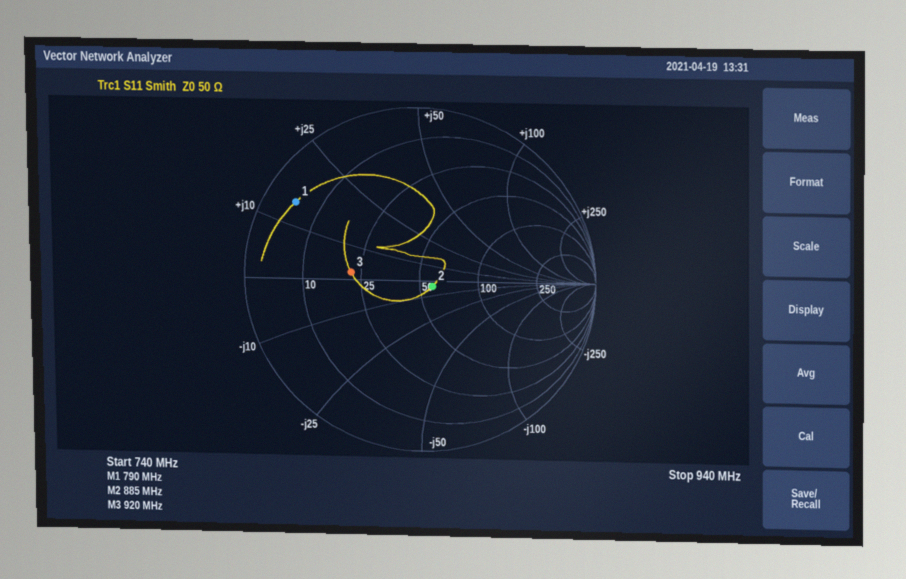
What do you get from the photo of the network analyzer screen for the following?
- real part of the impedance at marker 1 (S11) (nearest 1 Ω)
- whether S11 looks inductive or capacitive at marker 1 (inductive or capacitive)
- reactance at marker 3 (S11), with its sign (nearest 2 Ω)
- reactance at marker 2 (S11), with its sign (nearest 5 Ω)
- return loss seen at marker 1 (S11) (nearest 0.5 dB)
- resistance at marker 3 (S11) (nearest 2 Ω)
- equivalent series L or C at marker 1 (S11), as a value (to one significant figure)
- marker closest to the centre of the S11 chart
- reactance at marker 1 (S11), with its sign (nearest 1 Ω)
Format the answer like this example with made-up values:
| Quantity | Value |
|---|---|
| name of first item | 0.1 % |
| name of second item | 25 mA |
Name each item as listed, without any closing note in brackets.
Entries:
| Quantity | Value |
|---|---|
| real part of the impedance at marker 1 (S11) | 5 Ω |
| whether S11 looks inductive or capacitive at marker 1 | inductive |
| reactance at marker 3 (S11), with its sign | +2 Ω |
| reactance at marker 2 (S11), with its sign | -5 Ω |
| return loss seen at marker 1 (S11) | 1.5 dB |
| resistance at marker 3 (S11) | 22 Ω |
| equivalent series L or C at marker 1 (S11), as a value | 3 nH |
| marker closest to the centre of the S11 chart | marker 2 |
| reactance at marker 1 (S11), with its sign | +14 Ω |
